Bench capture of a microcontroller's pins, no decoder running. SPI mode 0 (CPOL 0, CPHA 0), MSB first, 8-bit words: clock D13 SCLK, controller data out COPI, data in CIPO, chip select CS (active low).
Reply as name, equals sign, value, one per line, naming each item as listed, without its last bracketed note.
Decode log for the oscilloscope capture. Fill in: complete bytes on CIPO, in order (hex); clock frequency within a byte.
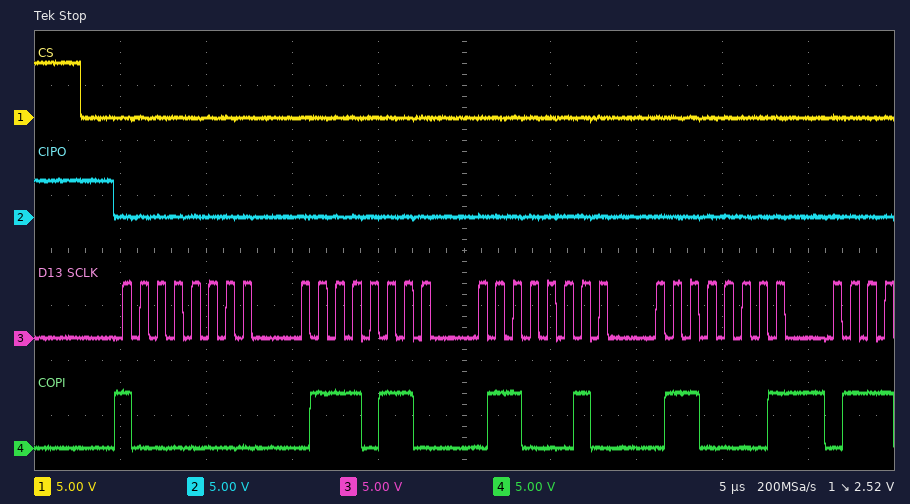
complete bytes on CIPO, in order = 00 00 00 00
clock frequency within a byte = 1 MHz
